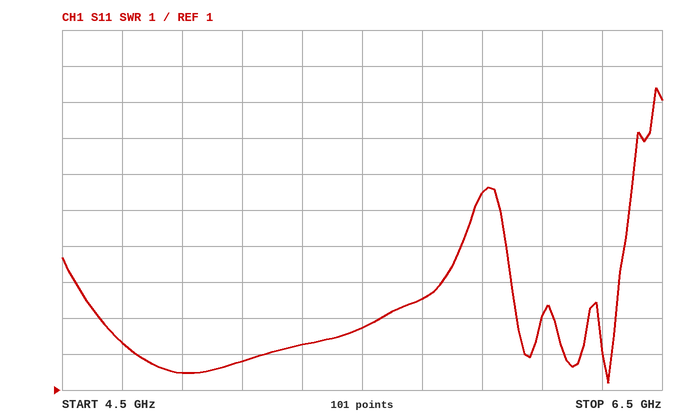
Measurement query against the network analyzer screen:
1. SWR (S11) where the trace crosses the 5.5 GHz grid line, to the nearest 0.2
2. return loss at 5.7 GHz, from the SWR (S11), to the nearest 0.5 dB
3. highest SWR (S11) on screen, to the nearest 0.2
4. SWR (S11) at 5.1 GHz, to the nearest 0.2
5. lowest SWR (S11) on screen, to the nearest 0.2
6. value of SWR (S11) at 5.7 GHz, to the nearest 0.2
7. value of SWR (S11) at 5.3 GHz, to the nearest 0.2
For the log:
2.8
5.0 dB
9.4
1.8
1.2
3.6
2.2
